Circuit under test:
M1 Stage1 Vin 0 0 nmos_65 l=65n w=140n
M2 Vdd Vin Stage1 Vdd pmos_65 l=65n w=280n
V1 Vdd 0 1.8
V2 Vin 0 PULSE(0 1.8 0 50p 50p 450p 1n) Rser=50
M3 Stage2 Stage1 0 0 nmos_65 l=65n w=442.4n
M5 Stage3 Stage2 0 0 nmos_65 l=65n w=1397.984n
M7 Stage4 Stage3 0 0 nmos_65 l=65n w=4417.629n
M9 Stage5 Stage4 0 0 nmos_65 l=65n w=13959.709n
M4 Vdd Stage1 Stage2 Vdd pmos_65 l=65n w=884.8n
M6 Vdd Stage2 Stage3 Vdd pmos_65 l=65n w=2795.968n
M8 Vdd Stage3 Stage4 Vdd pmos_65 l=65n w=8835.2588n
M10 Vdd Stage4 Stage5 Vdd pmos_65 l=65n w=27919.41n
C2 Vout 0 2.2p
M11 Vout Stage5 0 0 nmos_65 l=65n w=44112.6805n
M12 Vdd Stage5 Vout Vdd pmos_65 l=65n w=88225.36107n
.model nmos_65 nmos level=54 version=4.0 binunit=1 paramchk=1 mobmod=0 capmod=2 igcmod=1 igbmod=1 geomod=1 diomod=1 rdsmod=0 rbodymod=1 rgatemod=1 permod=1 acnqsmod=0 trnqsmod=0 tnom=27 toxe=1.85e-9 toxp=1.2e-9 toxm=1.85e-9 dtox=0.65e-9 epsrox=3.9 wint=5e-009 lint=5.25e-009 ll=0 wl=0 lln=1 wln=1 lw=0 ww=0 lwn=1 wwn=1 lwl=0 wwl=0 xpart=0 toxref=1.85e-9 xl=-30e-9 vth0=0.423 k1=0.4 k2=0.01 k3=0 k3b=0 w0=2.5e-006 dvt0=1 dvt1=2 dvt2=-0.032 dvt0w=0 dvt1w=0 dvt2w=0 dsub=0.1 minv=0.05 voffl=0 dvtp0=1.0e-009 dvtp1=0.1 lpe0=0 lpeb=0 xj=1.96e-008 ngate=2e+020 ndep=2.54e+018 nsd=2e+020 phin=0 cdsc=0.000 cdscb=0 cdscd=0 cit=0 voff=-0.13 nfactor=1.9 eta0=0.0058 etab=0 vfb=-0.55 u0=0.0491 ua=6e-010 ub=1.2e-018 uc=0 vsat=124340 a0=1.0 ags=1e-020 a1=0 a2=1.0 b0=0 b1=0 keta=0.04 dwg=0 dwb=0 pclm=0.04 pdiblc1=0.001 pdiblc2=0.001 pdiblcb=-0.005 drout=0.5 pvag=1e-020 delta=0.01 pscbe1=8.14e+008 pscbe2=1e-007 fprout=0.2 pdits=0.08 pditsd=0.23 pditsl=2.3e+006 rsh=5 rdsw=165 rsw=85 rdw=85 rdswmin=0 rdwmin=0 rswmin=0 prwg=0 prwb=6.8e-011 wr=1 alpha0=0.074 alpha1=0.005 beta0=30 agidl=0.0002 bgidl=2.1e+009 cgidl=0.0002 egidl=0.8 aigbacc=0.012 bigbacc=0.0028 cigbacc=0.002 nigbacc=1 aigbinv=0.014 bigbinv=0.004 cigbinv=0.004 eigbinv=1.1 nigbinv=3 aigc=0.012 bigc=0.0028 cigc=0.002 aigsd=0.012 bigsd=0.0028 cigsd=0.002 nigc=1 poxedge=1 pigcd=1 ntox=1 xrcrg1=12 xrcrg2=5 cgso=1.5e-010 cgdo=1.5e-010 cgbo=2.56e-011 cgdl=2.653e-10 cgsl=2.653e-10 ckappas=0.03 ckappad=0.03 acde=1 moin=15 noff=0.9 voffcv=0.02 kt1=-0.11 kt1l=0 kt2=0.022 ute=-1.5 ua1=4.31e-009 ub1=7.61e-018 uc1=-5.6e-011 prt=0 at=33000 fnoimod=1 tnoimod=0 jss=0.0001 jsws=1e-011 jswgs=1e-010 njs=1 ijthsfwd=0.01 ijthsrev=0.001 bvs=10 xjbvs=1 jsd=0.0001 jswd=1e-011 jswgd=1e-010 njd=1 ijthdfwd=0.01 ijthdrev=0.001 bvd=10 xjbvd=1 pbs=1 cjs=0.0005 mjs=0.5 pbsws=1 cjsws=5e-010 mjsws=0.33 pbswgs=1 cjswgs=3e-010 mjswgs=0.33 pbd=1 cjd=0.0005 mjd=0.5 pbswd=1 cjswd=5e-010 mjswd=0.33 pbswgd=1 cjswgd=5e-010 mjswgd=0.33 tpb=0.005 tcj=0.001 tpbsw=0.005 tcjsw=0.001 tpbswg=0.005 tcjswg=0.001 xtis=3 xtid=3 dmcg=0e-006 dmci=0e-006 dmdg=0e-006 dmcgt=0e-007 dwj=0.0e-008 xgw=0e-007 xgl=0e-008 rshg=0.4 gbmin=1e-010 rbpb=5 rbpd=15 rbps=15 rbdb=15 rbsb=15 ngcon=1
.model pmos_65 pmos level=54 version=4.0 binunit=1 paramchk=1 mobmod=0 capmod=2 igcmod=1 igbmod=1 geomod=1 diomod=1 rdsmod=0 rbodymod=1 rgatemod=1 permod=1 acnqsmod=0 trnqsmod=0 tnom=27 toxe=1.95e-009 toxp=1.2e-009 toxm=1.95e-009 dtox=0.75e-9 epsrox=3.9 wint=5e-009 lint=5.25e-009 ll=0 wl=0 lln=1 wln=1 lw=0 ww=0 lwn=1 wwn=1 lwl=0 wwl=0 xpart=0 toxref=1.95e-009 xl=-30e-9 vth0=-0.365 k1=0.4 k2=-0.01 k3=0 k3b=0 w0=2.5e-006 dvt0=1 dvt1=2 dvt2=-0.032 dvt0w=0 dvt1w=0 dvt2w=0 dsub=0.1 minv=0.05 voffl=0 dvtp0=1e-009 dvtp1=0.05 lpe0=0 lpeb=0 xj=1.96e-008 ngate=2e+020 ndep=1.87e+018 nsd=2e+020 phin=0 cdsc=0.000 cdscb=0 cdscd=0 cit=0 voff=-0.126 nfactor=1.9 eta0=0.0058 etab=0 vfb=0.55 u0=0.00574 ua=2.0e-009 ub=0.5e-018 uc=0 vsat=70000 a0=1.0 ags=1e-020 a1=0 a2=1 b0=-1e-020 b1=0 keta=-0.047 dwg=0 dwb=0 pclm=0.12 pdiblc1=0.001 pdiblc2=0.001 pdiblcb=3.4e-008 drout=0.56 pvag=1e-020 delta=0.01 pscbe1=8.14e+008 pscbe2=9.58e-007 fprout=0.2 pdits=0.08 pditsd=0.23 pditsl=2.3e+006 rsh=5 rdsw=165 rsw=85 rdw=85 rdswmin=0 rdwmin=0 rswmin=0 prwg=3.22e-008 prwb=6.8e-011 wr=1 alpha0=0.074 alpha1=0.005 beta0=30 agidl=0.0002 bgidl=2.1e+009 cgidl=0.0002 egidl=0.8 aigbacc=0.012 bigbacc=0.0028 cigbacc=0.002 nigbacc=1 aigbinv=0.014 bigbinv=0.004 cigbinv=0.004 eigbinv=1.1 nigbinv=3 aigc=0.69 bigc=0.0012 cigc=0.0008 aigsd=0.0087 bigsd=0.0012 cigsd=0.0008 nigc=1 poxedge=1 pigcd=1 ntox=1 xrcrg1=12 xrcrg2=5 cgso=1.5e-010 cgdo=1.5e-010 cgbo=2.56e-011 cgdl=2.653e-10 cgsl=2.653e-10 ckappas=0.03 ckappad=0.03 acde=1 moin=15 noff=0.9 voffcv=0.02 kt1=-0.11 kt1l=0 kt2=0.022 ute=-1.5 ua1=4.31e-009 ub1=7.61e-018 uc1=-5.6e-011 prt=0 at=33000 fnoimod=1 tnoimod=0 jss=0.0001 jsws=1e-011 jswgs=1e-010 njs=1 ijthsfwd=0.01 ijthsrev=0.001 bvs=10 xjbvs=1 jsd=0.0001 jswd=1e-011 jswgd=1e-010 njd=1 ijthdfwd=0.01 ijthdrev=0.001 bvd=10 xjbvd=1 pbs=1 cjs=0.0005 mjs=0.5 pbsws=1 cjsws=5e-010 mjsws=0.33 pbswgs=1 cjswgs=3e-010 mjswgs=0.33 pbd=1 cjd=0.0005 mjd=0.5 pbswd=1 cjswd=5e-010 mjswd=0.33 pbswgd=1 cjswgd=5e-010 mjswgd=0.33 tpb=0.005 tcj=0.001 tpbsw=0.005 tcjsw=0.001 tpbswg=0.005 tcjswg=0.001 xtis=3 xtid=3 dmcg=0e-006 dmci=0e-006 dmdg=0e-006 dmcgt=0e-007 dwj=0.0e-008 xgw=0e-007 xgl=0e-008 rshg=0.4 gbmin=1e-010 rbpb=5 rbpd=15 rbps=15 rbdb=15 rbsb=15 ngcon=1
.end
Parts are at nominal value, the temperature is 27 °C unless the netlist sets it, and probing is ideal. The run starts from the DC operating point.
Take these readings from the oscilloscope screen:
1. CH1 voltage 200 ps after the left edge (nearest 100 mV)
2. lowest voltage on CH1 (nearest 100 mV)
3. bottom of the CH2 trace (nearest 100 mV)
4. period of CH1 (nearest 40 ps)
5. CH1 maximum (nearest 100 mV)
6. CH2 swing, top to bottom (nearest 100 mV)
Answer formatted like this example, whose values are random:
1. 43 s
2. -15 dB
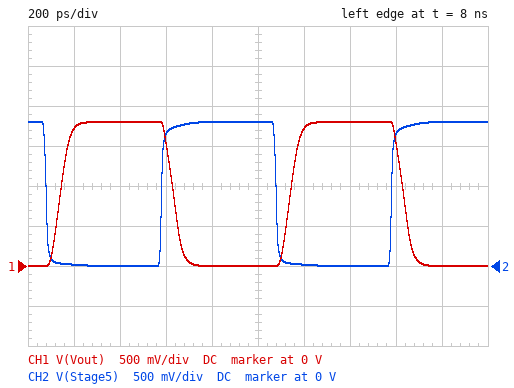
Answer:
1. 1.7 V
2. 0 V
3. 0 V
4. 1.00 ns
5. 1.8 V
6. 1.8 V
